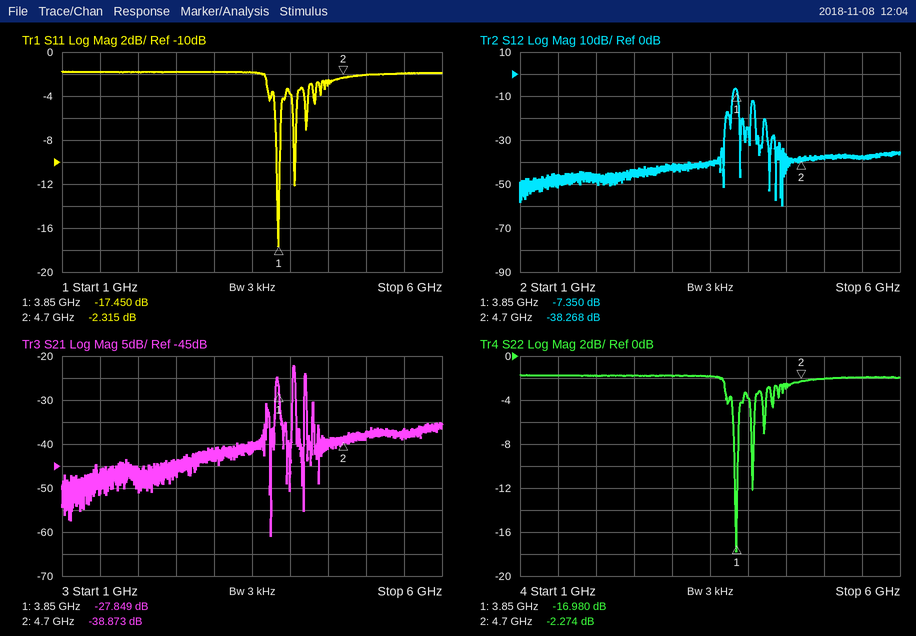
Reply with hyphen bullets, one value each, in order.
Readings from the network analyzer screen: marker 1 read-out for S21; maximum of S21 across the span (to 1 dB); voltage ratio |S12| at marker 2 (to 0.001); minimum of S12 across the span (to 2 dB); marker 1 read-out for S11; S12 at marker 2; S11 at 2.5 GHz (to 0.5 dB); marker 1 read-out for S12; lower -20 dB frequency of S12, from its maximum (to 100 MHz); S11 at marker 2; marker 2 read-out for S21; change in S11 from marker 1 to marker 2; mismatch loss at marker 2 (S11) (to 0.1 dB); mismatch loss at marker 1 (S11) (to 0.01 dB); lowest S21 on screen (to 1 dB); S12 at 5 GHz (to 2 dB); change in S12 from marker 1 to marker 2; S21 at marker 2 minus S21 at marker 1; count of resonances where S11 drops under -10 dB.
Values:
- -27.849 dB
- -22 dB
- 0.012
- -60 dB
- -17.450 dB
- -38.268 dB
- -2.0 dB
- -7.350 dB
- 3.7 GHz
- -2.315 dB
- -38.873 dB
- 15.135 dB
- 3.8 dB
- 0.08 dB
- -61 dB
- -38 dB
- -30.918 dB
- -11.024 dB
- 2
